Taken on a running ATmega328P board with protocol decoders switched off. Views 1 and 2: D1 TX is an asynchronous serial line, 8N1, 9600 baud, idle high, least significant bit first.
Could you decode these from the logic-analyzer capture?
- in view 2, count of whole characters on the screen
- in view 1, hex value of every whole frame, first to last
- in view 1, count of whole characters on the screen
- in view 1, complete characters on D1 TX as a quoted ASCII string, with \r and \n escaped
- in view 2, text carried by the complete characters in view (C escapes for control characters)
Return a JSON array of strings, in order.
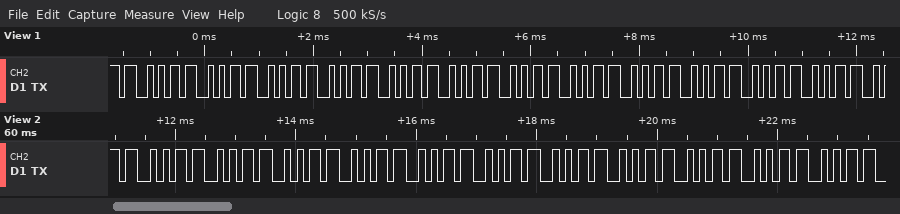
["11", "0x53 0x53 0x53 0x53 0x53 0x53 0x53 0x53 0x53 0x53 0x53 0x53", "12", "\"SSSSSSSSSSSS\"", "\"SSSSSSSSSSS\""]
